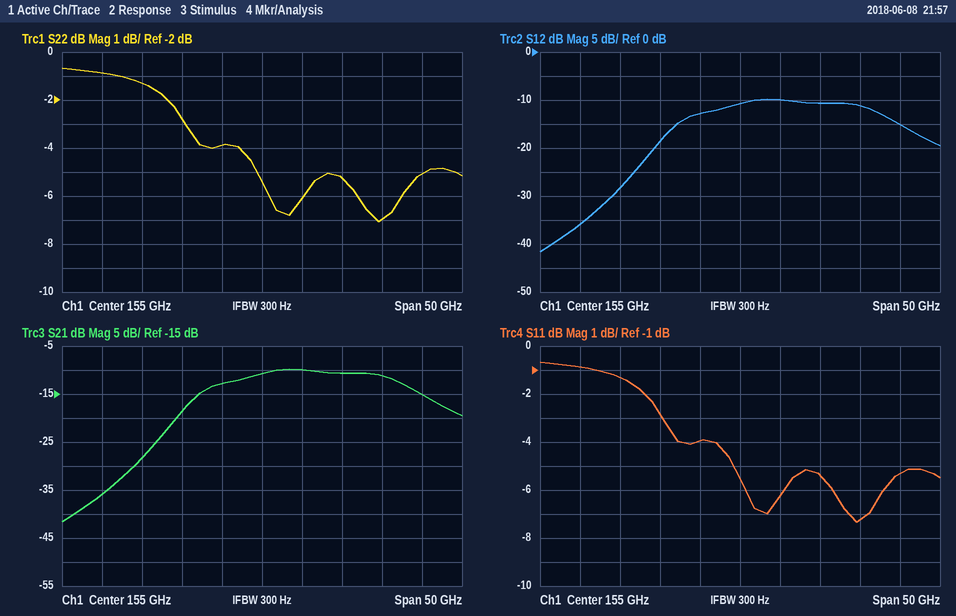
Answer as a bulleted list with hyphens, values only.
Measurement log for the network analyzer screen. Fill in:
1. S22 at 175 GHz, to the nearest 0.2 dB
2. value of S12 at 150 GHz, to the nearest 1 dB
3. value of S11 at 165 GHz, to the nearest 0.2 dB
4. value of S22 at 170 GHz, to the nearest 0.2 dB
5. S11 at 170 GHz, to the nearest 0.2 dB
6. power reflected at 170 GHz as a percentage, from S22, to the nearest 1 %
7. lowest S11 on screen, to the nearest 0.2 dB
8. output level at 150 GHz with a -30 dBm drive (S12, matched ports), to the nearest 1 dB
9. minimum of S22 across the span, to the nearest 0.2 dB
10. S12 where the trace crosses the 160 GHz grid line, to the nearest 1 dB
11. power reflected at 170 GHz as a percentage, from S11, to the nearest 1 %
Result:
- -5.0 dB
- -13 dB
- -5.4 dB
- -7.0 dB
- -7.2 dB
- 20 %
- -7.4 dB
- -43 dBm
- -7.0 dB
- -10 dB
- 19 %
